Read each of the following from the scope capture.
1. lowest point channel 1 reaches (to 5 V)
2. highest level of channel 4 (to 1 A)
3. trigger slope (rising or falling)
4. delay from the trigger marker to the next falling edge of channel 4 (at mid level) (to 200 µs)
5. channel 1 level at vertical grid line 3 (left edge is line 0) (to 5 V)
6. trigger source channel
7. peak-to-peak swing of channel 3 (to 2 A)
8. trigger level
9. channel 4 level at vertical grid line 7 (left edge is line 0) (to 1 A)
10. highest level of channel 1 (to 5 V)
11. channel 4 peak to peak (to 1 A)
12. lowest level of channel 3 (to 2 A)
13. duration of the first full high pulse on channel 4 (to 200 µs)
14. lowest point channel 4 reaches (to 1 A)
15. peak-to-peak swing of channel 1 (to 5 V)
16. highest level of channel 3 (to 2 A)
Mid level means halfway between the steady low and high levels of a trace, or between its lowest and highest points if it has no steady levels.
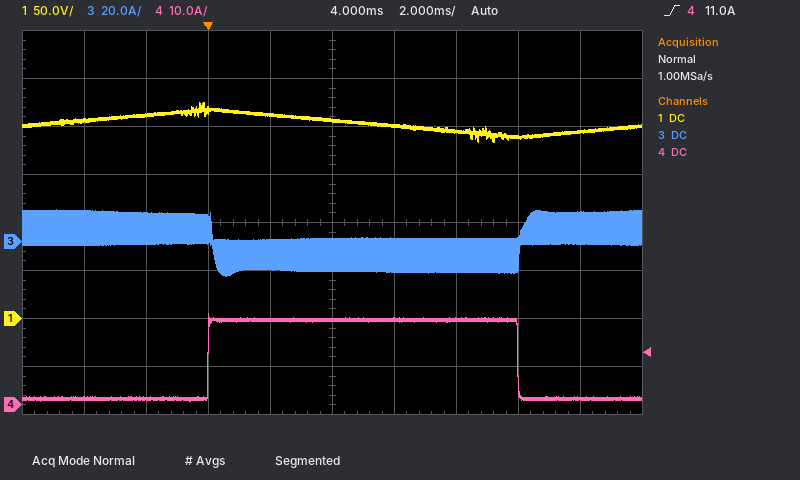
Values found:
185 V
19 A
rising
10.0 ms
215 V
channel 4
28 A
11.0 A
18 A
225 V
18 A
-14 A
10.0 ms
1 A
40 V
14 A
